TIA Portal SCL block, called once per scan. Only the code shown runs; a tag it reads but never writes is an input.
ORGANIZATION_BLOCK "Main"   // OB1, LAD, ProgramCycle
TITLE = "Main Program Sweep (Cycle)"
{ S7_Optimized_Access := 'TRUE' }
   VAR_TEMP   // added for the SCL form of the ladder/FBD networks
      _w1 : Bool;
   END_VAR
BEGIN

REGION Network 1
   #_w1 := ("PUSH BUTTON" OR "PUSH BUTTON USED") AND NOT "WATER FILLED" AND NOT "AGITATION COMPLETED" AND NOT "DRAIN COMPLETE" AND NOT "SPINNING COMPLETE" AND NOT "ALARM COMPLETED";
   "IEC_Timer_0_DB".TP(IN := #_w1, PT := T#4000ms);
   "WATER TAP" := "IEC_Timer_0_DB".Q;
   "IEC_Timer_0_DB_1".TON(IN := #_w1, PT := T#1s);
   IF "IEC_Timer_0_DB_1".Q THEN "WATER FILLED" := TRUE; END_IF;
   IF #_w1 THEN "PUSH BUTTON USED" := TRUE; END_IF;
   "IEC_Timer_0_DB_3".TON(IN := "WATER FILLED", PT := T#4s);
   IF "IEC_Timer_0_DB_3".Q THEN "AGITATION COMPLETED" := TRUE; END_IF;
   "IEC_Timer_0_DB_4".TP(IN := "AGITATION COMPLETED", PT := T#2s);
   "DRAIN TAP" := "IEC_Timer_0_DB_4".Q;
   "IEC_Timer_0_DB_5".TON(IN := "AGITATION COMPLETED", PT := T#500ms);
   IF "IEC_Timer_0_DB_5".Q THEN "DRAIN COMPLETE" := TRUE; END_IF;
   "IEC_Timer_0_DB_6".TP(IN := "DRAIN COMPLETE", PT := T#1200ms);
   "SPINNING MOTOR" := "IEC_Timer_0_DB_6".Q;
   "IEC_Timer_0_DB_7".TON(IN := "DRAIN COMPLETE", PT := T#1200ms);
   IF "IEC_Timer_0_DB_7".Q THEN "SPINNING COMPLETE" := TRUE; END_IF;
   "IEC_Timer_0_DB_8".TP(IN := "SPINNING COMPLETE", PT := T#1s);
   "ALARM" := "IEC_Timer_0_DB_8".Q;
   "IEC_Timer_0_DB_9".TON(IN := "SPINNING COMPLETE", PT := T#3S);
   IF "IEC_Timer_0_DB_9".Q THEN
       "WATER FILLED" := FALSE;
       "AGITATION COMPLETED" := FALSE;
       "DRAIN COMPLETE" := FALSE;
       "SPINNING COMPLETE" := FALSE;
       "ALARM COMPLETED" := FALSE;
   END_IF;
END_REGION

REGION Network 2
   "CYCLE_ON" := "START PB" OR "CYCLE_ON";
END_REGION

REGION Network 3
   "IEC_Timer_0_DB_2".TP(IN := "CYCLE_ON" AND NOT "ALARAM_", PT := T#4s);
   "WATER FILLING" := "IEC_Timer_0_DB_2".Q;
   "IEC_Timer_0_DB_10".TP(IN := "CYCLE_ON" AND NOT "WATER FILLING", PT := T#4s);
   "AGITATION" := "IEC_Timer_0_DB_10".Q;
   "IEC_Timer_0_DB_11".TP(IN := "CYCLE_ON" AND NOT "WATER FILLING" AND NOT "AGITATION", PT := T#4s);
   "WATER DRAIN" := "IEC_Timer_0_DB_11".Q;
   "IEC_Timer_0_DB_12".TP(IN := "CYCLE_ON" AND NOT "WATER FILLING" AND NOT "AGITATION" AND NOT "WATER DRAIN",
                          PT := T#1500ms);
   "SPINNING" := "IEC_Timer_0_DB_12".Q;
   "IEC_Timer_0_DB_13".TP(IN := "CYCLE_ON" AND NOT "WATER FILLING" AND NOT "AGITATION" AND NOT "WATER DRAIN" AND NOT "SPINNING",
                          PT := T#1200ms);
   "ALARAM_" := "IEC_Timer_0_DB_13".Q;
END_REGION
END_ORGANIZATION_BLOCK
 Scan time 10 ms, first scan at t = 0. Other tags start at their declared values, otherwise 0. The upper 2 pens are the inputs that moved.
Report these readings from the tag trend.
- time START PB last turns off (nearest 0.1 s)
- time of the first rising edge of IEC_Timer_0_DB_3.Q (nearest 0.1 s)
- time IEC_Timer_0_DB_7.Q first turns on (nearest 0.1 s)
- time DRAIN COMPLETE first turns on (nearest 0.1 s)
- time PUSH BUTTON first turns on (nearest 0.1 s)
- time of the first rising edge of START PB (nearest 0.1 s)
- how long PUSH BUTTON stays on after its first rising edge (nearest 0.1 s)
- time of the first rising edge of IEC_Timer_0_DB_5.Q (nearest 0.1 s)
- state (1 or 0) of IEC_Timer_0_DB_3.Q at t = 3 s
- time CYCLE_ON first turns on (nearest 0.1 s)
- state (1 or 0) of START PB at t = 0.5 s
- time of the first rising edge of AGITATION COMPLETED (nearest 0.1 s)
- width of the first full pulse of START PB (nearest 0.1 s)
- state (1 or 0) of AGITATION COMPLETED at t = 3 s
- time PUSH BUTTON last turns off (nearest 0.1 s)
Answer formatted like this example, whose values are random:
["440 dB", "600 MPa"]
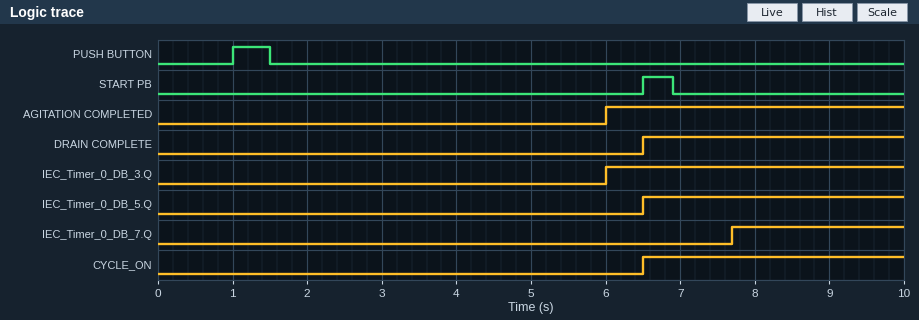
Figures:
["6.9 s", "6.0 s", "7.7 s", "6.5 s", "1.0 s", "6.5 s", "0.5 s", "6.5 s", "0", "6.5 s", "0", "6.0 s", "0.4 s", "0", "1.5 s"]
